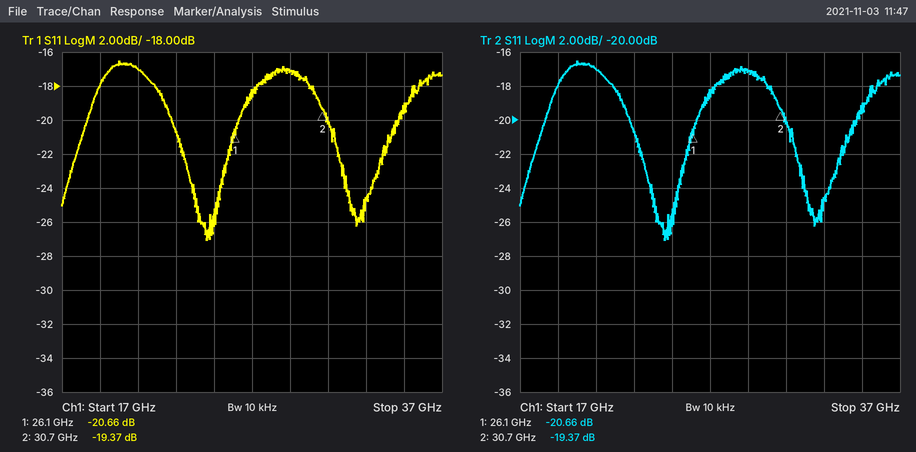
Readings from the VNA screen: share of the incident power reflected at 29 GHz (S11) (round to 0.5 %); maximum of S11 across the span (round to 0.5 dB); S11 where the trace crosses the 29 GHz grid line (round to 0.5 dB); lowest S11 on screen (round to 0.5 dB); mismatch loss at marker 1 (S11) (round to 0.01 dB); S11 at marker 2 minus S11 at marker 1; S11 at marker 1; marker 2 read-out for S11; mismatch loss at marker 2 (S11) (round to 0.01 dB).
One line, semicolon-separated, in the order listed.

2.0 %; -16.5 dB; -17.0 dB; -27.0 dB; 0.04 dB; 1.29 dB; -20.66 dB; -19.37 dB; 0.05 dB
